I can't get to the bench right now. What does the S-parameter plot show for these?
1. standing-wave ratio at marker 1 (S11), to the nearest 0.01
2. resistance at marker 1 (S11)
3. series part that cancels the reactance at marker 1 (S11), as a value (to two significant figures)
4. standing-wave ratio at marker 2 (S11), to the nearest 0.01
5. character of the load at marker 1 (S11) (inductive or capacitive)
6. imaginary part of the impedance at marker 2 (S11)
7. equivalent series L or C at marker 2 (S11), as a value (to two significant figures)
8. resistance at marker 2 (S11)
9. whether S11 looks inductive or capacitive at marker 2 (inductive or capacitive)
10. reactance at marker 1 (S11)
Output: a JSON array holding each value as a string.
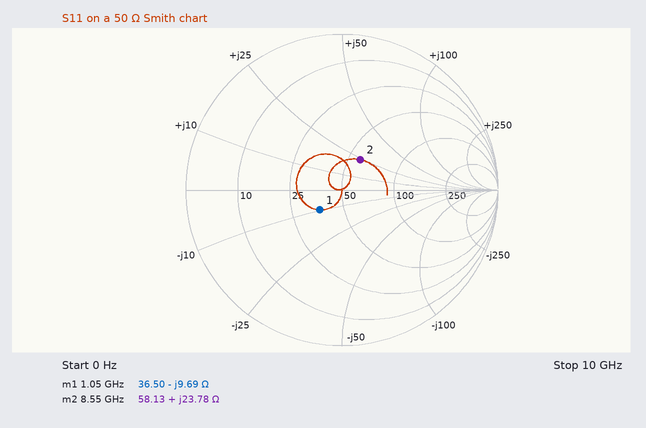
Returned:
["1.47", "36.50 Ω", "1.5 nH", "1.59", "capacitive", "+23.78 Ω", "440 pH", "58.13 Ω", "inductive", "-9.69 Ω"]
